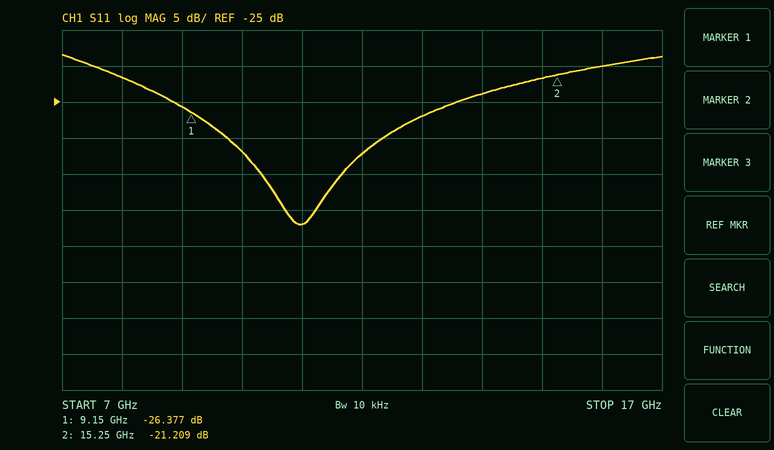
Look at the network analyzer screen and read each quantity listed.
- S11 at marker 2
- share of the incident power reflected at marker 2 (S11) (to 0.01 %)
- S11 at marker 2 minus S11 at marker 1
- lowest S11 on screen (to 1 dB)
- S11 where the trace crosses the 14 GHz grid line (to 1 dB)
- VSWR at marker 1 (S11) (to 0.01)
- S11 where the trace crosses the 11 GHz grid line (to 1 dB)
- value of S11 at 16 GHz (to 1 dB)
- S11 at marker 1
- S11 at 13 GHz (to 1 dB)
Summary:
-21.209 dB
0.76 %
5.168 dB
-42 dB
-24 dB
1.10
-42 dB
-20 dB
-26.377 dB
-27 dB
